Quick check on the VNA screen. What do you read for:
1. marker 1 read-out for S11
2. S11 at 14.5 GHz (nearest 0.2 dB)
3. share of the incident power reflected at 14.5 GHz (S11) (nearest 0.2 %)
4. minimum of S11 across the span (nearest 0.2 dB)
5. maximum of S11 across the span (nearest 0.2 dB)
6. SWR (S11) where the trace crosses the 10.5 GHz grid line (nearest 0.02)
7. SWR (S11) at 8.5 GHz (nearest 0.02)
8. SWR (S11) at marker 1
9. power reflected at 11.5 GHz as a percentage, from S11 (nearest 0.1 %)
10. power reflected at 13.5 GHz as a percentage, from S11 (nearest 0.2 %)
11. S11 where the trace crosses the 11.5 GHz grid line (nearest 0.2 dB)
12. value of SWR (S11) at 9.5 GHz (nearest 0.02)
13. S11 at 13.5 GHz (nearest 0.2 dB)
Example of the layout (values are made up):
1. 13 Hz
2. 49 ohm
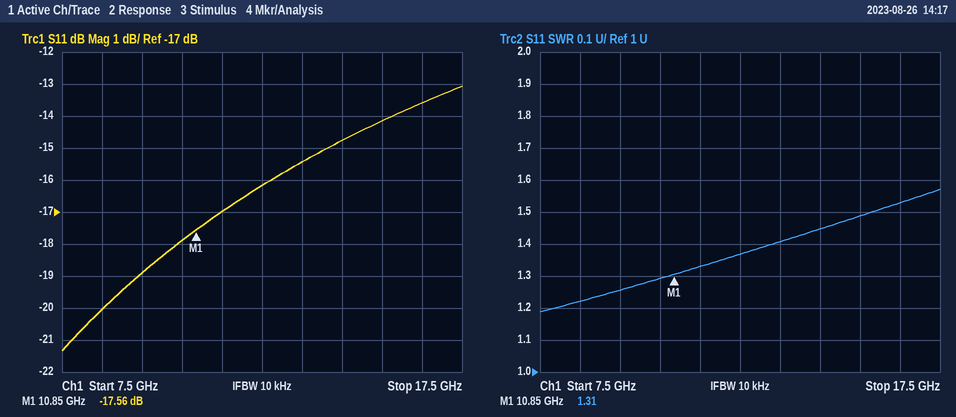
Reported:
1. -17.56 dB
2. -14.8 dB
3. 3.4 %
4. -21.4 dB
5. -13.0 dB
6. 1.30
7. 1.22
8. 1.31
9. 2.0 %
10. 2.8 %
11. -17.0 dB
12. 1.26
13. -15.4 dB
